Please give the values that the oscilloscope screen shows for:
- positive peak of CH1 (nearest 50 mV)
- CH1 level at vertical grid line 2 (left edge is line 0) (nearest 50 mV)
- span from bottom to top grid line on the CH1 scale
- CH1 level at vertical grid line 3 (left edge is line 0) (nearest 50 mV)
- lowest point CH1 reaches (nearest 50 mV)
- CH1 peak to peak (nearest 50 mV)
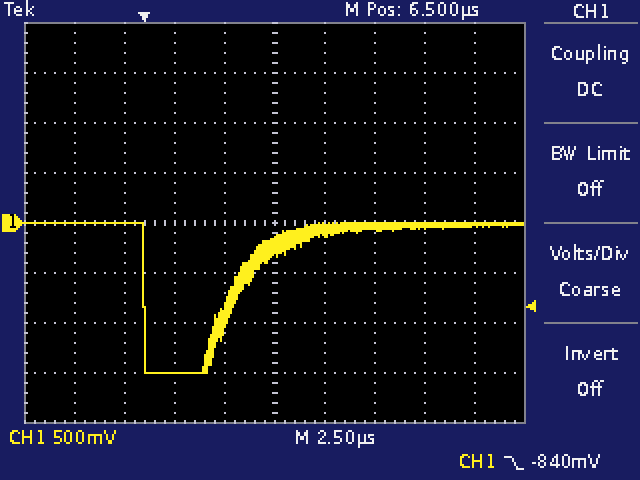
0 mV
0 mV
4 V
-1.50 V
-1.50 V
1.50 V
